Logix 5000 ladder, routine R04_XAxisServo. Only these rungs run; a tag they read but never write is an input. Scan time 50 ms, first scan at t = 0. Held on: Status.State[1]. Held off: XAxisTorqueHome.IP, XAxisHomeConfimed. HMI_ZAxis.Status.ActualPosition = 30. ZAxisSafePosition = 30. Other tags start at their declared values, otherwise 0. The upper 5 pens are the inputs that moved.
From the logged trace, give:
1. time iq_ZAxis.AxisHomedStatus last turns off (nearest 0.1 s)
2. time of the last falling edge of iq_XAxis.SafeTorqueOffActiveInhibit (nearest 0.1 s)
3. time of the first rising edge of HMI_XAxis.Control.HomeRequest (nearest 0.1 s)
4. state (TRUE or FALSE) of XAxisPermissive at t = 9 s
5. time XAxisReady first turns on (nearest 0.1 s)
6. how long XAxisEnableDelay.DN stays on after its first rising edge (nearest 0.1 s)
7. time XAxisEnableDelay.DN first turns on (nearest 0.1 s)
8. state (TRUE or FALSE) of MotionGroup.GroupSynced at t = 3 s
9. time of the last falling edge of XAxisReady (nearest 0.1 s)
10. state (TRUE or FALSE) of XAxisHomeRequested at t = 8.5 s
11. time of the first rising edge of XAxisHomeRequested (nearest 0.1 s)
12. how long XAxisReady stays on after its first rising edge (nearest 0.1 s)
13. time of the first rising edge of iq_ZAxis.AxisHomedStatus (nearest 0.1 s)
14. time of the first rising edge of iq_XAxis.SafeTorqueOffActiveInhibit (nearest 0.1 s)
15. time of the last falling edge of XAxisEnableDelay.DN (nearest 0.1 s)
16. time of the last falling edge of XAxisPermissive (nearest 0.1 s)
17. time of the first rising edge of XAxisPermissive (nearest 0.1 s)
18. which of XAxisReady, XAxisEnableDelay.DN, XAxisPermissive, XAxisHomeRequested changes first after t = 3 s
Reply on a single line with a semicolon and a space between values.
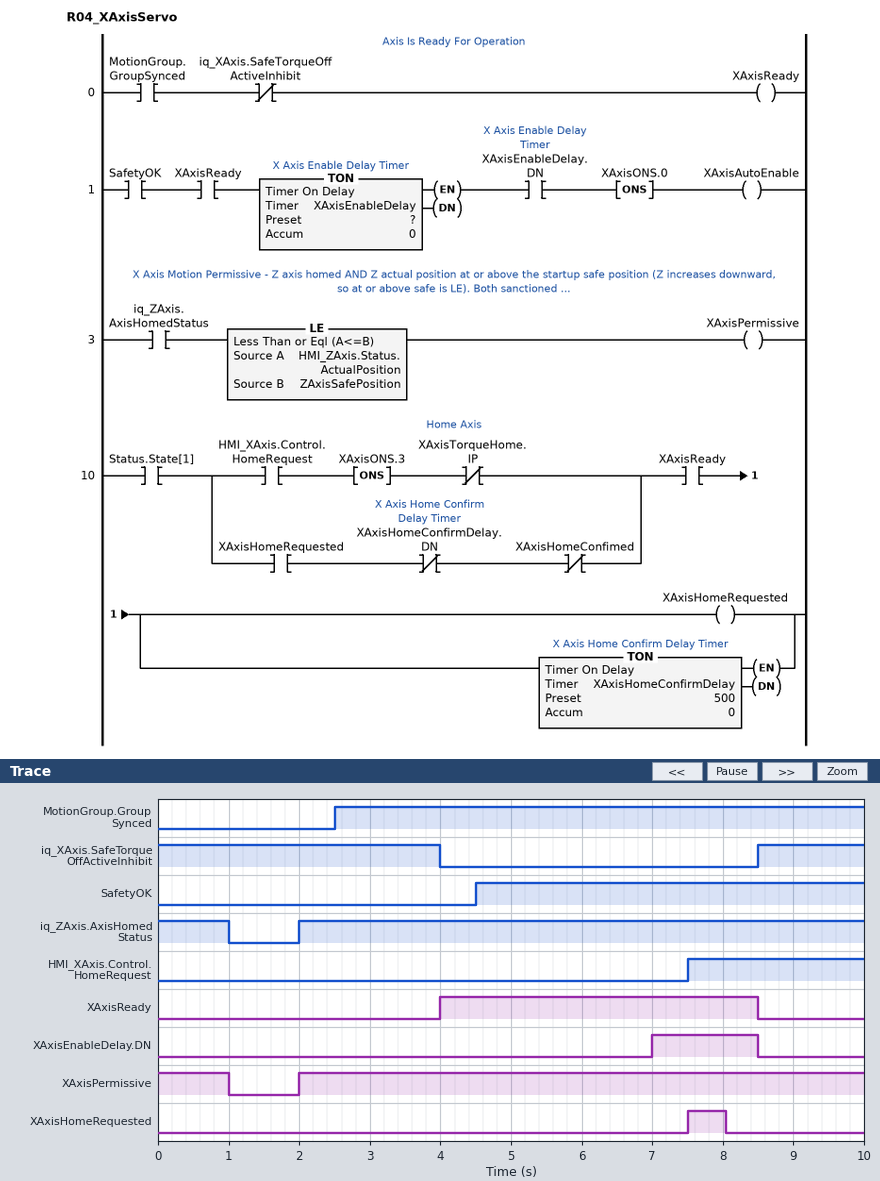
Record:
1.0 s; 4.0 s; 7.5 s; TRUE; 4.0 s; 1.5 s; 7.0 s; TRUE; 8.5 s; FALSE; 7.5 s; 4.5 s; 2.0 s; 8.5 s; 8.5 s; 1.0 s; 2.0 s; XAxisReady
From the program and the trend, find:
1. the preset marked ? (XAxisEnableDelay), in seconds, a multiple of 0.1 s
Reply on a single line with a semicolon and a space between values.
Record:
2.5 s
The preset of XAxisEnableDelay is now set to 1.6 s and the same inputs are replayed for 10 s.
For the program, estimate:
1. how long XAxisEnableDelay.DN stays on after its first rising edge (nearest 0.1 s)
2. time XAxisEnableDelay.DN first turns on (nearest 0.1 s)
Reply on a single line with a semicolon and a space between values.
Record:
2.4 s; 6.1 s
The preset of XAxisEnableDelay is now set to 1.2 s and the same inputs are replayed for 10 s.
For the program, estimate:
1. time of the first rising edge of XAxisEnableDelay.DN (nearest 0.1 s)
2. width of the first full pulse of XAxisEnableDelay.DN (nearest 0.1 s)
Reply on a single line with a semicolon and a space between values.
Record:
5.7 s; 2.8 s
